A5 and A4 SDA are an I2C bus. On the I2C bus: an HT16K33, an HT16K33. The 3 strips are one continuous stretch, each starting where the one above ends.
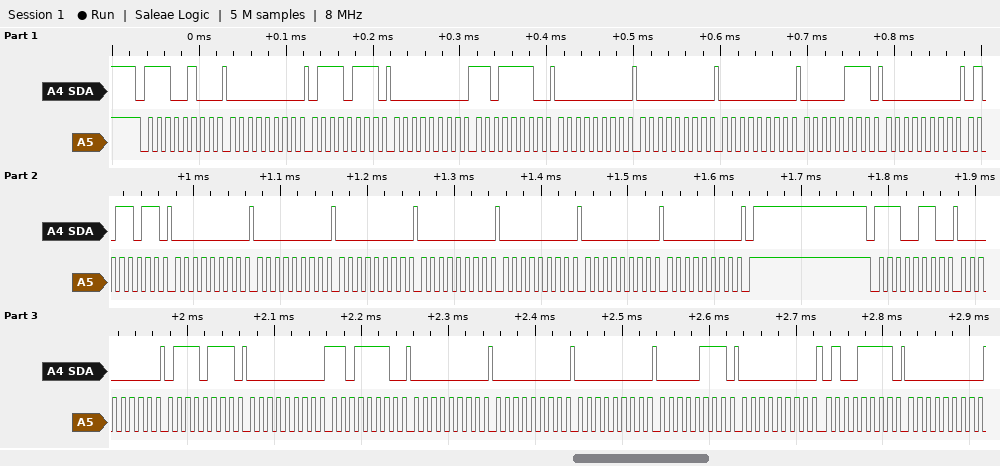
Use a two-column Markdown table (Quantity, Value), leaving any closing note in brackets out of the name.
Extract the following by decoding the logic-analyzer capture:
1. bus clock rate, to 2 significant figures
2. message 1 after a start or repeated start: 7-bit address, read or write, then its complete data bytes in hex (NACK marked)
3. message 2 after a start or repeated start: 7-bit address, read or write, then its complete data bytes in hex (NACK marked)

| Quantity | Value |
|---|---|
| bus clock rate, to 2 significant figures | 100 kHz |
| message 1 after a start or repeated start: 7-bit address, read or write, then its complete data bytes in hex | 0x72 write: 00 77 00 DE 00 00 00 07 00 5B 00 00 00 00 00 00 00 |
| message 2 after a start or repeated start: 7-bit address, read or write, then its complete data bytes in hex | 0x73 write: 00 77 00 DE 00 00 00 07 00 4F 00 |
